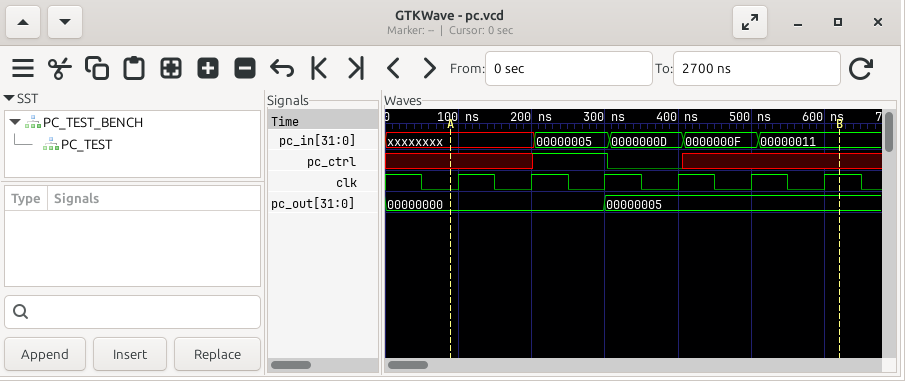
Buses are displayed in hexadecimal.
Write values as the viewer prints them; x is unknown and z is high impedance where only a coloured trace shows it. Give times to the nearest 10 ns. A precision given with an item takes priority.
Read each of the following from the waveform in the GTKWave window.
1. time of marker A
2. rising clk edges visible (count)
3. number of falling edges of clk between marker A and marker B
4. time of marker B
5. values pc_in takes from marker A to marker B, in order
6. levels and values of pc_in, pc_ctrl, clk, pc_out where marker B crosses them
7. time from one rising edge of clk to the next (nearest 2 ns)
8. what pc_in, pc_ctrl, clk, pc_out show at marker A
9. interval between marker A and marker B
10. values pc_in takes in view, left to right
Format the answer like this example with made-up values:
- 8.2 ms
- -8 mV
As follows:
- 90 ns
- 6
- 5
- 620 ns
- xxxxxxxx, 00000005, 0000000D, 0000000F, 00000011
- pc_in=00000011, pc_ctrl=x, clk=1, pc_out=00000005
- 100 ns
- pc_in=xxxxxxxx, pc_ctrl=x, clk=0, pc_out=00000000
- 530 ns
- xxxxxxxx, 00000005, 0000000D, 0000000F, 00000011
